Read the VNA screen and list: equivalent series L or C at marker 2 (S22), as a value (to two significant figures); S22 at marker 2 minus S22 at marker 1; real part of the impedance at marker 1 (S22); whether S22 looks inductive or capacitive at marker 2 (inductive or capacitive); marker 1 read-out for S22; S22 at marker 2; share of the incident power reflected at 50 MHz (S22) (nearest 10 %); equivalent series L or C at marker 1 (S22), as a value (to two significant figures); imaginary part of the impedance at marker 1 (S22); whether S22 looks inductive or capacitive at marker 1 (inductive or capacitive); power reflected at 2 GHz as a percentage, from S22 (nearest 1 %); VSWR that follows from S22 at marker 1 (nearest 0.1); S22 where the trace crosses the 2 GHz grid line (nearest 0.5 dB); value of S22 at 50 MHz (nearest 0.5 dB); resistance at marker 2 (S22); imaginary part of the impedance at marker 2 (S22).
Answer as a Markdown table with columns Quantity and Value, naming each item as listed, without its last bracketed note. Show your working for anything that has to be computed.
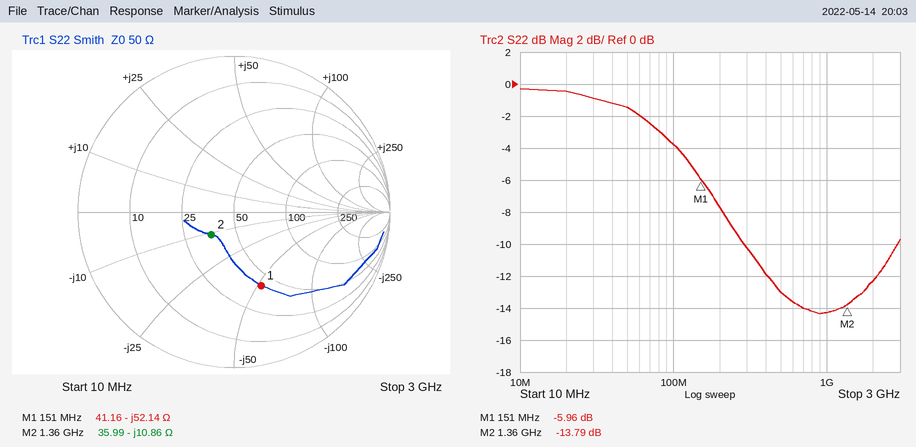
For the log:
| Quantity | Value |
|---|---|
| equivalent series L or C at marker 2 (S22), as a value | C = 1/(2π × 1.36 GHz × 10.86 Ω) ≈ 11 pF |
| S22 at marker 2 minus S22 at marker 1 | -13.79 − (-5.96) = -7.83 dB |
| real part of the impedance at marker 1 | 41.16 Ω |
| whether S22 looks inductive or capacitive at marker 2 | capacitive |
| marker 1 read-out for S22 | -5.96 dB |
| S22 at marker 2 | -13.79 dB |
| share of the incident power reflected at 50 MHz (S22) | 10^(-1.5/10) ≈ 70.8 %, so 70 % to the nearest 10 % |
| equivalent series L or C at marker 1 (S22), as a value | C = 1/(2π × 151 MHz × 52.14 Ω) ≈ 20 pF |
| imaginary part of the impedance at marker 1 | -52.14 Ω |
| whether S22 looks inductive or capacitive at marker 1 | capacitive |
| power reflected at 2 GHz as a percentage, from S22 | 10^(-12.5/10) ≈ 6 % |
| VSWR that follows from S22 at marker 1 | (1 + 0.5035)/(1 − 0.5035) ≈ 3.0 |
| S22 where the trace crosses the 2 GHz grid line | -12.5 dB |
| value of S22 at 50 MHz | -1.5 dB |
| resistance at marker 2 | 35.99 Ω |
| imaginary part of the impedance at marker 2 | -10.86 Ω |
